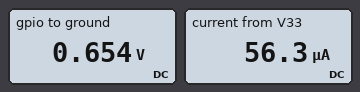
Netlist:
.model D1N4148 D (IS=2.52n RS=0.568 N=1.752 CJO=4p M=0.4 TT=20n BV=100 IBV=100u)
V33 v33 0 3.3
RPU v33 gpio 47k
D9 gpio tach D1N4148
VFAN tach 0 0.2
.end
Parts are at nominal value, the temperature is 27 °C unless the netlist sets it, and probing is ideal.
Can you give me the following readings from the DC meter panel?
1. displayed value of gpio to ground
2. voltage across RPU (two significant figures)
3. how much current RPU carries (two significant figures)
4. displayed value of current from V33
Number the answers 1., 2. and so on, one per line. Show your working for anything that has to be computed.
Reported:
1. 0.654 V
2. 3.3 V - 654 mV = 2.6 V
3. (3.3 V - 654 mV) / 47 kΩ = 56 µA
4. 56.3 µA
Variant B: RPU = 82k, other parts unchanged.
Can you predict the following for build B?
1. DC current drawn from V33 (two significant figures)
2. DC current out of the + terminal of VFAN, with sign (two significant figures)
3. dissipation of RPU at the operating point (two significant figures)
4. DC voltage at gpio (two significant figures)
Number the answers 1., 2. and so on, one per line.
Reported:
1. 33 µA
2. -33 µA
3. 87 µW
4. 630 mV
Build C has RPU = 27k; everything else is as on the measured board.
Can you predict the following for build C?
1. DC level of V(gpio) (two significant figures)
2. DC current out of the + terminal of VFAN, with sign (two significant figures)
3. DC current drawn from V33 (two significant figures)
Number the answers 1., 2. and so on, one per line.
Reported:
1. 680 mV
2. -97 µA
3. 97 µA
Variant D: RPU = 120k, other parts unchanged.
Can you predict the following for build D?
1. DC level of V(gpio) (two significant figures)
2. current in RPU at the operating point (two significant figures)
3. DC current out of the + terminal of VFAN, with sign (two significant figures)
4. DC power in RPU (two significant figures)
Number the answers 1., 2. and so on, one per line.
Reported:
1. 610 mV
2. 22 µA
3. -22 µA
4. 60 µW
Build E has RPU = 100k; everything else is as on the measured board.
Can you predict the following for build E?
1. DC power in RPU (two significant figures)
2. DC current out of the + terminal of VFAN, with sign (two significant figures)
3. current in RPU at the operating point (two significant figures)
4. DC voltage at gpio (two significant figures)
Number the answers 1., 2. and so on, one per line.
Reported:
1. 72 µW
2. -27 µA
3. 27 µA
4. 620 mV
